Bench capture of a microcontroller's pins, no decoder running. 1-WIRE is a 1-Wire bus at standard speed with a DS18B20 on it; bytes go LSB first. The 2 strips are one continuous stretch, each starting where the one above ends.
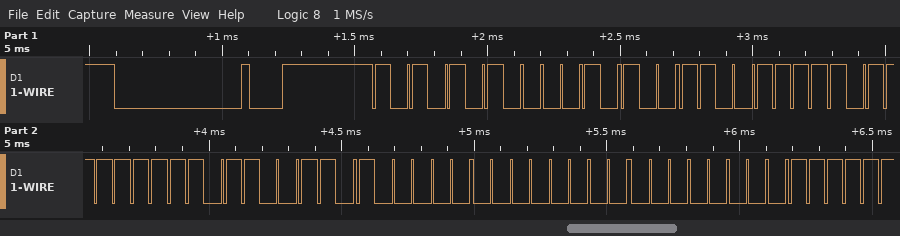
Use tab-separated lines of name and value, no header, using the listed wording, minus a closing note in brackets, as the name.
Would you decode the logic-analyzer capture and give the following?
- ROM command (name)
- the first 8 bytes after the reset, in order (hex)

ROM command	Match ROM
the first 8 bytes after the reset, in order	55 28 F3 FD 9B 05 00 00
